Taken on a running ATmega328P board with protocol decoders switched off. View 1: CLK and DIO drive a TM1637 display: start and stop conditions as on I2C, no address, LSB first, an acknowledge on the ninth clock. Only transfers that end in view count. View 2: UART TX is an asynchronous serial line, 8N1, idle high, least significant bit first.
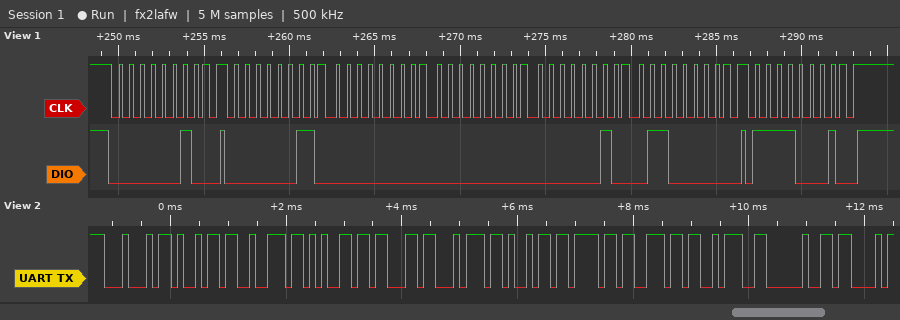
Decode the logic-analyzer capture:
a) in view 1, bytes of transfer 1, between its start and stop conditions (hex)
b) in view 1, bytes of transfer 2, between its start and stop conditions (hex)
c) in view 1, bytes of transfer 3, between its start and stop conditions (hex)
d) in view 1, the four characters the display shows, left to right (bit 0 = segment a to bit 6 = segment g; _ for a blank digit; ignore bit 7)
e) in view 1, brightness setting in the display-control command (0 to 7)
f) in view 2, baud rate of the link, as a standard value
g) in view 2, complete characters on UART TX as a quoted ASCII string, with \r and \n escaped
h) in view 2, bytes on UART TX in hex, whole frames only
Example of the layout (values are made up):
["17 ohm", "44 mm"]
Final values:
["40", "C0 00 00 40 06", "8F", "__-1", "7", "9600 baud", "\"Direction: C\"", "44 69 72 65 63 74 69 6F 6E 3A 20 43"]
